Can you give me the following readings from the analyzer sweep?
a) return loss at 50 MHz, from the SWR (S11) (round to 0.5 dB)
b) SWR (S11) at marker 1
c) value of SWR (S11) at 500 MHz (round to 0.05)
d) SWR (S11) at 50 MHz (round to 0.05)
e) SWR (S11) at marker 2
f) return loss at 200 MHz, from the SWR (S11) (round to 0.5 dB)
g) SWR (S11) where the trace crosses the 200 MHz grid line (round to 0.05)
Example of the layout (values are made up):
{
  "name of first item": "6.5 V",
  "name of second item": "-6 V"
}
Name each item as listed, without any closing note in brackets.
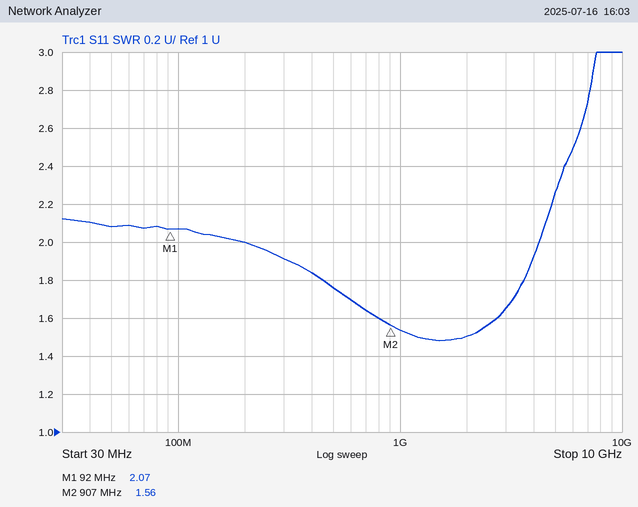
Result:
{
  "return loss at 50 MHz, from the SWR (S11)": "9.0 dB",
  "SWR (S11) at marker 1": "2.07",
  "value of SWR (S11) at 500 MHz": "1.75",
  "SWR (S11) at 50 MHz": "2.10",
  "SWR (S11) at marker 2": "1.56",
  "return loss at 200 MHz, from the SWR (S11)": "9.5 dB",
  "SWR (S11) where the trace crosses the 200 MHz grid line": "2.00"
}
